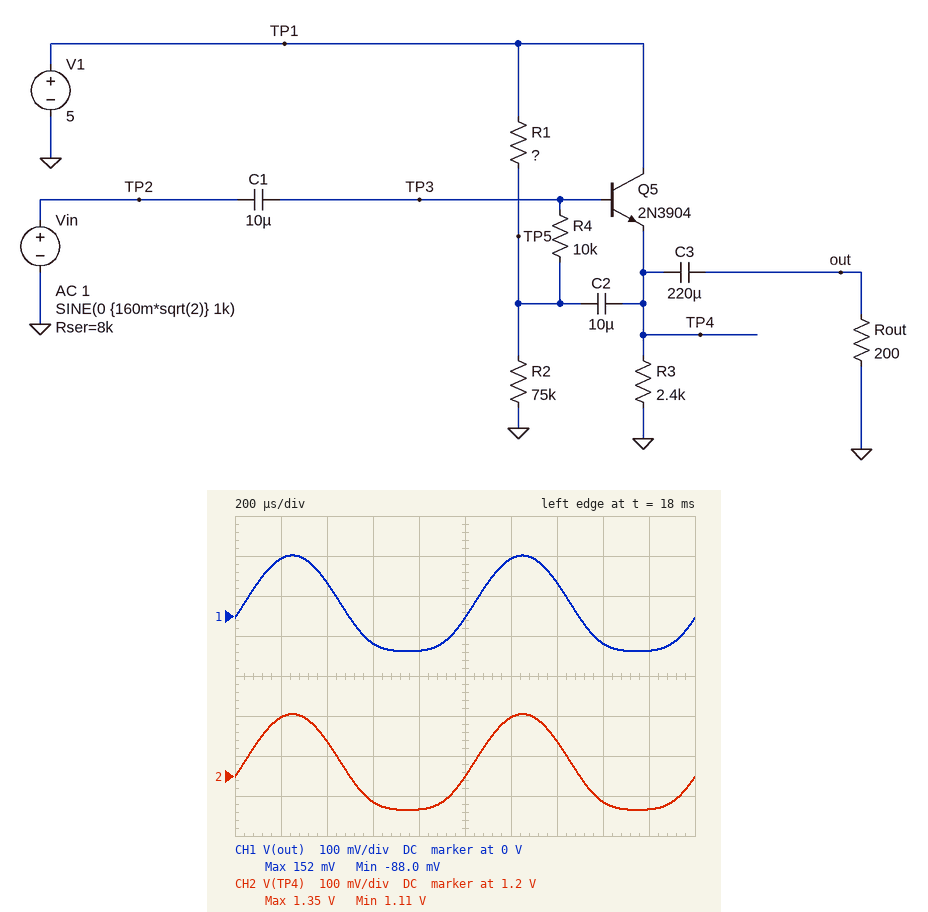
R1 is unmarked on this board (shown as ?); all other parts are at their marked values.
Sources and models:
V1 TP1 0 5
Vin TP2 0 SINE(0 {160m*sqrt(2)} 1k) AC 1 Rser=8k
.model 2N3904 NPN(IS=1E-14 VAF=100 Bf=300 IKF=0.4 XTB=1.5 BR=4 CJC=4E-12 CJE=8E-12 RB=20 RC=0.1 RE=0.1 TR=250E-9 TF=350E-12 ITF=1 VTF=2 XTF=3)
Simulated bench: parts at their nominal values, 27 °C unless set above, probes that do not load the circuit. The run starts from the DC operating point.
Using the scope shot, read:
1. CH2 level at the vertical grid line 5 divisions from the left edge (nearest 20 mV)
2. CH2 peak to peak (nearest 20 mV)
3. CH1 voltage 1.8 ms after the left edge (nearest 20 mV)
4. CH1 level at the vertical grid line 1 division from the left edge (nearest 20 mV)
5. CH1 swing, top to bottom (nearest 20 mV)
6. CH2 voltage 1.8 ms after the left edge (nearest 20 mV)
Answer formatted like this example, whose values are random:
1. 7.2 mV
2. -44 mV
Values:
1. 1.20 V
2. 240 mV
3. -80 mV
4. 140 mV
5. 240 mV
6. 1.12 V
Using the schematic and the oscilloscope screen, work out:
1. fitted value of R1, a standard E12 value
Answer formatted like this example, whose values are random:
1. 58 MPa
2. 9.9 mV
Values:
1. 120 kΩ
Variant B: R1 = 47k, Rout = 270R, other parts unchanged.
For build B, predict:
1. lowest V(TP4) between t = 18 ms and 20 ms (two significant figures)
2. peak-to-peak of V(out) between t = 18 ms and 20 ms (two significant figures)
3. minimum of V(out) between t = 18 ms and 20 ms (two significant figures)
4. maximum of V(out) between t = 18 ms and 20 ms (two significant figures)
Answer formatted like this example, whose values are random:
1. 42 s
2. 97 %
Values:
1. 2.1 V
2. 340 mV
3. -160 mV
4. 180 mV
